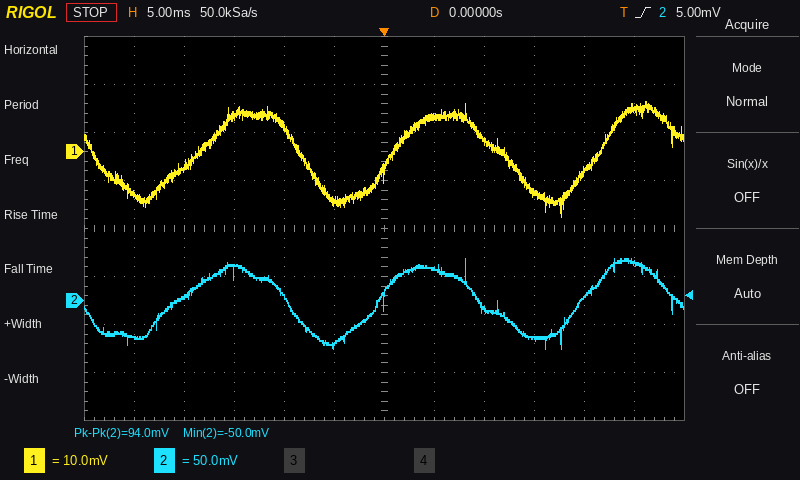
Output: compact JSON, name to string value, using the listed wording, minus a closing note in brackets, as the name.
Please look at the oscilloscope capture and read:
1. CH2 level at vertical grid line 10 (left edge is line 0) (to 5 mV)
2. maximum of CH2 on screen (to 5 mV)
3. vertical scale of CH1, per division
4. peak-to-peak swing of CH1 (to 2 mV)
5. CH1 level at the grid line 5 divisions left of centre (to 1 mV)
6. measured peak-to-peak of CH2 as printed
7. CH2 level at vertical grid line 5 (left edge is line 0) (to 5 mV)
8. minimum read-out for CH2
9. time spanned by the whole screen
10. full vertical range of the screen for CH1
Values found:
{"CH2 level at vertical grid line 10 (left edge is line 0)": "5 mV", "maximum of CH2 on screen": "45 mV", "vertical scale of CH1, per division": "10 mV", "peak-to-peak swing of CH1": "24 mV", "CH1 level at the grid line 5 divisions left of centre": "-9 mV", "measured peak-to-peak of CH2 as printed": "94.0 mV", "CH2 level at vertical grid line 5 (left edge is line 0)": "-45 mV", "minimum read-out for CH2": "-50.0 mV", "time spanned by the whole screen": "60 ms", "full vertical range of the screen for CH1": "80 mV"}
